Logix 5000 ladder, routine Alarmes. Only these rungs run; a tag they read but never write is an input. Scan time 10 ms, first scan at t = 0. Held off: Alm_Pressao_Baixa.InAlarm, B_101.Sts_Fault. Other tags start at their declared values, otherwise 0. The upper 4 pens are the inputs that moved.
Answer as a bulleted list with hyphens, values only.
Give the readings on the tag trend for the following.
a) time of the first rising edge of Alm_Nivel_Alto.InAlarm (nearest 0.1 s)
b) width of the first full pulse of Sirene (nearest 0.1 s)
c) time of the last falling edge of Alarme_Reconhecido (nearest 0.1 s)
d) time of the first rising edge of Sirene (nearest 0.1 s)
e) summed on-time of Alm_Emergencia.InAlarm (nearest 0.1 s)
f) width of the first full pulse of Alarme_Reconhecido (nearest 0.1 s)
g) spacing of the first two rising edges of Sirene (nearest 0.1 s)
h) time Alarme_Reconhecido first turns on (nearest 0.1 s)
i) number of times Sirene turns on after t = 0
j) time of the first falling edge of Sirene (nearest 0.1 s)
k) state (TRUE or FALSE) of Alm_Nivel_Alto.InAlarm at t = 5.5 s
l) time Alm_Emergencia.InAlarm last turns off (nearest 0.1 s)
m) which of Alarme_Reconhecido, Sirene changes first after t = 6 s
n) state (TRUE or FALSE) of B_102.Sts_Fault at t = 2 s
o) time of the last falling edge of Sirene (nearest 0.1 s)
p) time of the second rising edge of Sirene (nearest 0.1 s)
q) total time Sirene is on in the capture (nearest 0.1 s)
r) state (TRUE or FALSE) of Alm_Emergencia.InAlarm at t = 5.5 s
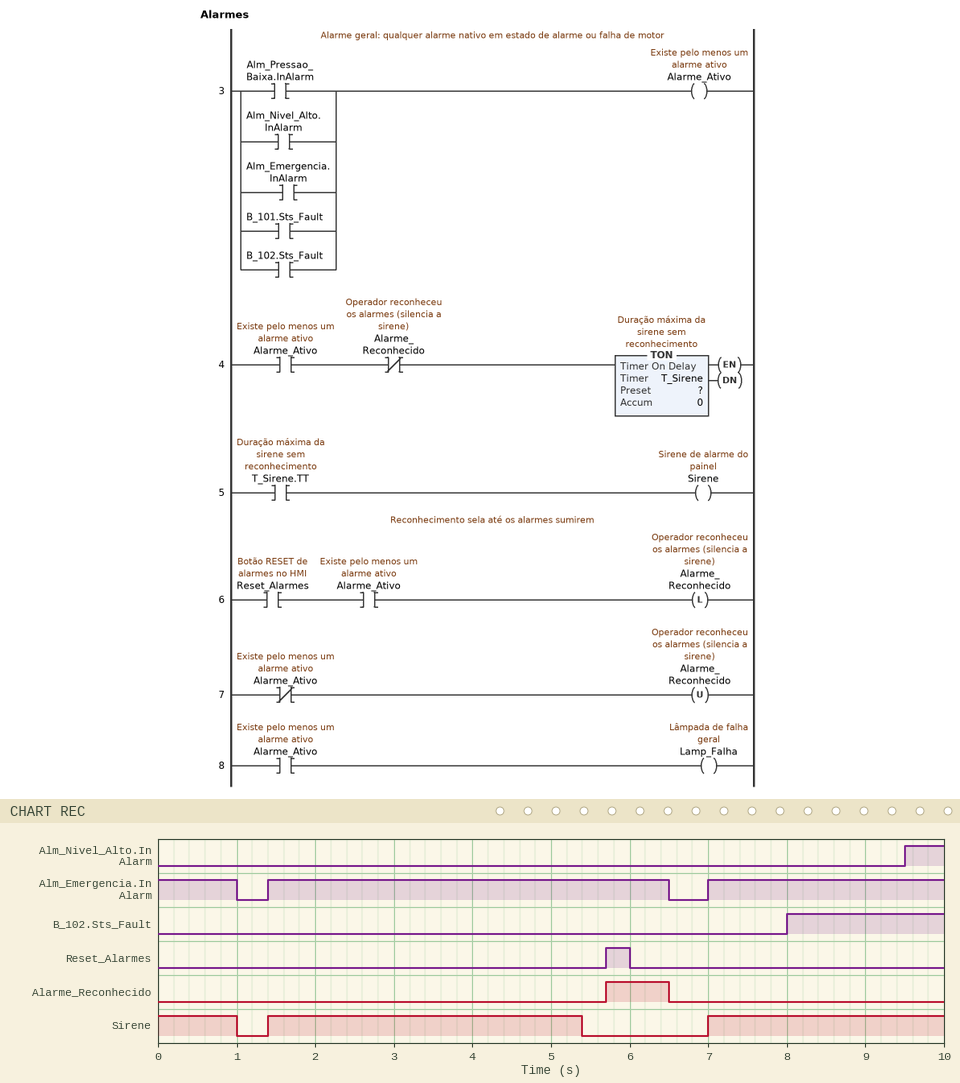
- 9.5 s
- 4.0 s
- 6.5 s
- 1.4 s
- 9.1 s
- 0.8 s
- 5.6 s
- 5.7 s
- 2
- 1.0 s
- FALSE
- 6.5 s
- Alarme_Reconhecido
- FALSE
- 5.4 s
- 7.0 s
- 8.0 s
- TRUE
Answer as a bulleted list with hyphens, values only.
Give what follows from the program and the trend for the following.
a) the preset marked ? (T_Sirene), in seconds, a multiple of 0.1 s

- 4.0 s
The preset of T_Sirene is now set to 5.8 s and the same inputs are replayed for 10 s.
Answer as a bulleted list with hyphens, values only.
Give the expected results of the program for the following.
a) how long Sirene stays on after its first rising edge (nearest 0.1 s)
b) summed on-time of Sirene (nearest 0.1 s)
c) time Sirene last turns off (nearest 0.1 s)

- 4.3 s
- 8.3 s
- 5.7 s
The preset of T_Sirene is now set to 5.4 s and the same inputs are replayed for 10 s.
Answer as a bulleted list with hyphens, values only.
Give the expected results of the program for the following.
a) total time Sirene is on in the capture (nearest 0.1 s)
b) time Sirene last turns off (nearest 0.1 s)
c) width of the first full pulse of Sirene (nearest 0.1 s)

- 8.3 s
- 5.7 s
- 4.3 s
